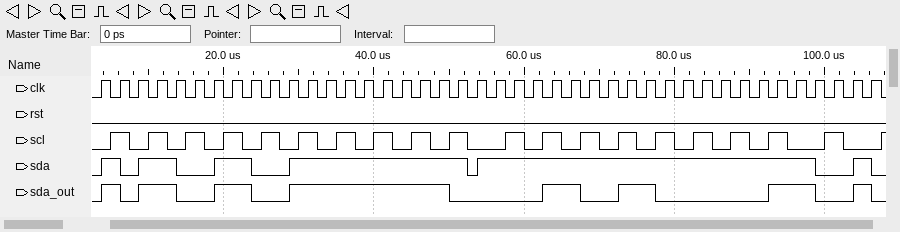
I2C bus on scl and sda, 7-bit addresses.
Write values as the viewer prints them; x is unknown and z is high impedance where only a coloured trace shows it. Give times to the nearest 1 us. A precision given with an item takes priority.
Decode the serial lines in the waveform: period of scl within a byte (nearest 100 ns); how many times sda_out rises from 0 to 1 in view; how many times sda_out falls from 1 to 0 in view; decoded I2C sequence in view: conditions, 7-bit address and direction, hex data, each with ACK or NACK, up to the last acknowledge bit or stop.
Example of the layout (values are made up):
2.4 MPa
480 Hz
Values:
5000 ns
8
8
start, address 57 read NACK, FF ACK
